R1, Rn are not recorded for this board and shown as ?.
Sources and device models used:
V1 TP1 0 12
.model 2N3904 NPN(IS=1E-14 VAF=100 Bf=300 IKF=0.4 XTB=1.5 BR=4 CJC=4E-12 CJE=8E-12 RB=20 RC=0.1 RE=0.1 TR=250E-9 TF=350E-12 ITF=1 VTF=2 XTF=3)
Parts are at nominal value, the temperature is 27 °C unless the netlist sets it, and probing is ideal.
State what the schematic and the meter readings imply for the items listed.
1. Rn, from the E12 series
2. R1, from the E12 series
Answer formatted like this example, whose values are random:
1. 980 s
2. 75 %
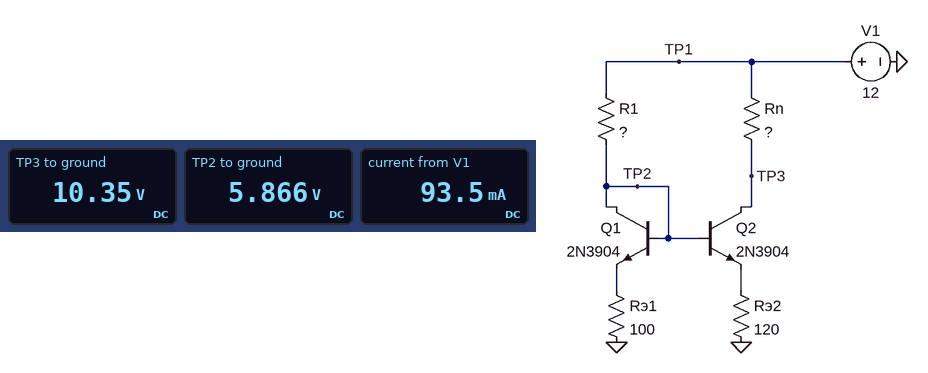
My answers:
1. 39 Ω
2. 120 Ω
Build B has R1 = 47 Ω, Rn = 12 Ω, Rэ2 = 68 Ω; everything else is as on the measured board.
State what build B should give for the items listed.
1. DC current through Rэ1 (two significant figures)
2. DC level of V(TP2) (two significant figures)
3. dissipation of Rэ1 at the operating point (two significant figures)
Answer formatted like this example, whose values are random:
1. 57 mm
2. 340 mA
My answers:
1. 76 mA
2. 8.4 V
3. 580 mW
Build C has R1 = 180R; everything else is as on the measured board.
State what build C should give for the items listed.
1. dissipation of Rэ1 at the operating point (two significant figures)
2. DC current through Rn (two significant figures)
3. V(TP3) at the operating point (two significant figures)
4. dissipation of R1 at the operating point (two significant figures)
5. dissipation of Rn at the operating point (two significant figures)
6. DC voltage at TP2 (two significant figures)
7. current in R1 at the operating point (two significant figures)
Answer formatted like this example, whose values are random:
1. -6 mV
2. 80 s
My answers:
1. 160 mW
2. 33 mA
3. 11 V
4. 290 mW
5. 43 mW
6. 4.8 V
7. 40 mA
